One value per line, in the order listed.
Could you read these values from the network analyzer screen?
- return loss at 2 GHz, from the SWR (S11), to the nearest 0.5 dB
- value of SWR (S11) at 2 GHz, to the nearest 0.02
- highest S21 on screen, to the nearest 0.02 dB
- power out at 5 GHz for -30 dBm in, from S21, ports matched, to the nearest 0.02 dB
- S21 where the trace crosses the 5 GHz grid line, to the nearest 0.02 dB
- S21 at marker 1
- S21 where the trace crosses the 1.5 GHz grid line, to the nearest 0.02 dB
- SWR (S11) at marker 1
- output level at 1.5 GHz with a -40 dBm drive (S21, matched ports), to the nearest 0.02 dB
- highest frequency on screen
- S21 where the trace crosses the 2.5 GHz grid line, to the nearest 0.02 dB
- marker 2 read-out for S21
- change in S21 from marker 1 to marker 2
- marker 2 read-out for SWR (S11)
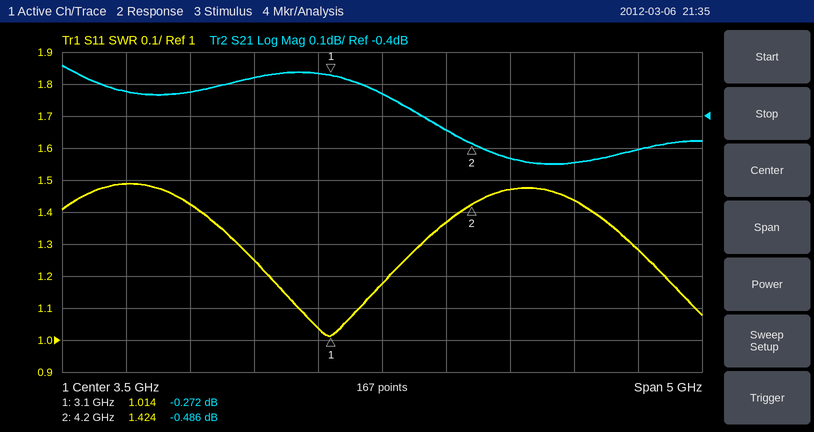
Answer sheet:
15.0 dB
1.42
-0.24 dB
-30.54 dBm
-0.54 dB
-0.272 dB
-0.32 dB
1.014
-40.32 dBm
6 GHz
-0.28 dB
-0.486 dB
-0.214 dB
1.424
